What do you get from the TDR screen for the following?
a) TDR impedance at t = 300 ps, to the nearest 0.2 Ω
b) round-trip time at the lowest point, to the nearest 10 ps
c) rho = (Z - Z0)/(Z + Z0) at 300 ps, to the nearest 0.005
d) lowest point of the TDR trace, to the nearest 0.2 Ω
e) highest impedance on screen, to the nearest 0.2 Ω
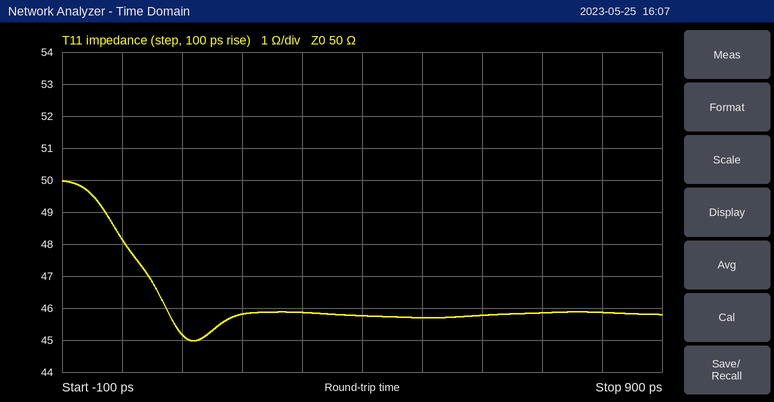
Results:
45.8 Ω
120 ps
-0.045
45.0 Ω
50.0 Ω
